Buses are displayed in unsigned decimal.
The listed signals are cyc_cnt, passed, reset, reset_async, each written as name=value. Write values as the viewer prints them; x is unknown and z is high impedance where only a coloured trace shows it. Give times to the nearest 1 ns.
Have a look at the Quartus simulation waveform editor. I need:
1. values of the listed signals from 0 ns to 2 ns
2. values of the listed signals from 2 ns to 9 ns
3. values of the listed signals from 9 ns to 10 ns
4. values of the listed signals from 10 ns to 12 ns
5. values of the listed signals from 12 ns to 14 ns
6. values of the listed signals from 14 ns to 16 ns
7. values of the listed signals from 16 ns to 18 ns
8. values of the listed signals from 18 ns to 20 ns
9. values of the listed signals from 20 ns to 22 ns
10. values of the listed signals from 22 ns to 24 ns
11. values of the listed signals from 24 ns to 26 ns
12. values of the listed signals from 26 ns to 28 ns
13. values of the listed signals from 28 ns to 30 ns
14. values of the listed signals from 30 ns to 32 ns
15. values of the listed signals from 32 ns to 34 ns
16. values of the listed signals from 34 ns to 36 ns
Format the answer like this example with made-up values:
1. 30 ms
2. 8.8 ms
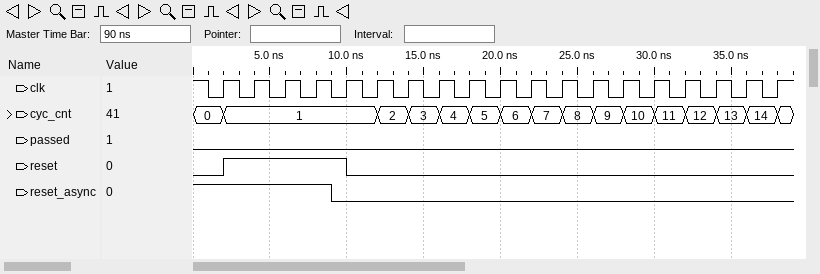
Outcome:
1. cyc_cnt=0, passed=0, reset=0, reset_async=1
2. cyc_cnt=1, passed=0, reset=1, reset_async=1
3. cyc_cnt=1, passed=0, reset=1, reset_async=0
4. cyc_cnt=1, passed=0, reset=0, reset_async=0
5. cyc_cnt=2, passed=0, reset=0, reset_async=0
6. cyc_cnt=3, passed=0, reset=0, reset_async=0
7. cyc_cnt=4, passed=0, reset=0, reset_async=0
8. cyc_cnt=5, passed=0, reset=0, reset_async=0
9. cyc_cnt=6, passed=0, reset=0, reset_async=0
10. cyc_cnt=7, passed=0, reset=0, reset_async=0
11. cyc_cnt=8, passed=0, reset=0, reset_async=0
12. cyc_cnt=9, passed=0, reset=0, reset_async=0
13. cyc_cnt=10, passed=0, reset=0, reset_async=0
14. cyc_cnt=11, passed=0, reset=0, reset_async=0
15. cyc_cnt=12, passed=0, reset=0, reset_async=0
16. cyc_cnt=13, passed=0, reset=0, reset_async=0
